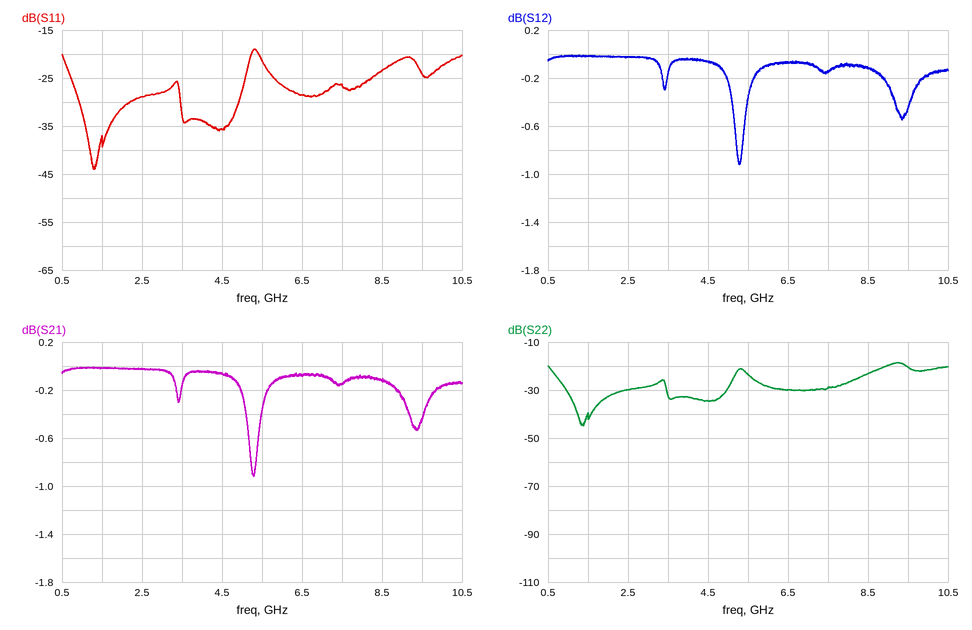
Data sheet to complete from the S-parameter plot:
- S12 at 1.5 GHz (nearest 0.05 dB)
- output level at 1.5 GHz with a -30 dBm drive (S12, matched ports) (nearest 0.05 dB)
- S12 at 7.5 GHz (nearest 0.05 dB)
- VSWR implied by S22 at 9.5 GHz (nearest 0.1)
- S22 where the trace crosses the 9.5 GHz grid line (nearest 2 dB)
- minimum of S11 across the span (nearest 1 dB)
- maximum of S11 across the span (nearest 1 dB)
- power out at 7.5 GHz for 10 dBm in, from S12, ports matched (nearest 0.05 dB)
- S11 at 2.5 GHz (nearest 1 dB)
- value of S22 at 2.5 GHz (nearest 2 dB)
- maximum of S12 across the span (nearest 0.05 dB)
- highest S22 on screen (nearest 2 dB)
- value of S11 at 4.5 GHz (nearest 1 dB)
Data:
0.00 dB
-30.00 dBm
-0.15 dB
1.2
-20 dB
-44 dB
-19 dB
9.85 dBm
-29 dB
-30 dB
0.00 dB
-18 dB
-36 dB
